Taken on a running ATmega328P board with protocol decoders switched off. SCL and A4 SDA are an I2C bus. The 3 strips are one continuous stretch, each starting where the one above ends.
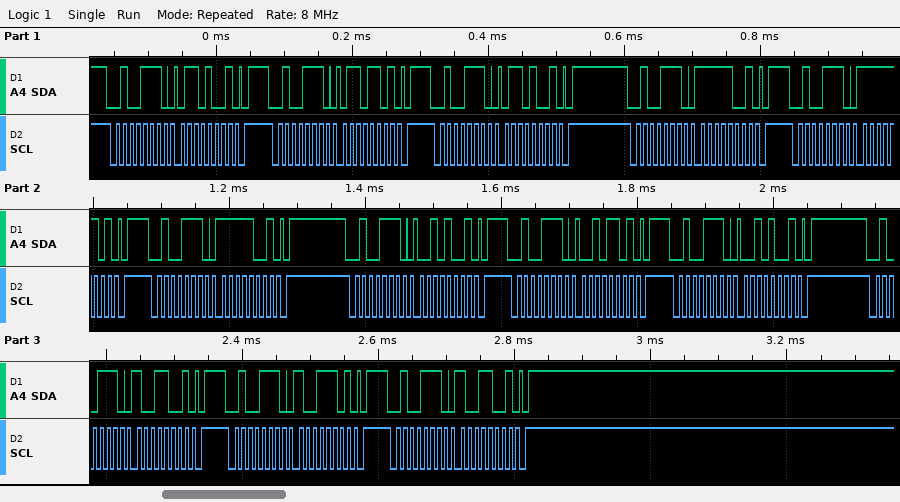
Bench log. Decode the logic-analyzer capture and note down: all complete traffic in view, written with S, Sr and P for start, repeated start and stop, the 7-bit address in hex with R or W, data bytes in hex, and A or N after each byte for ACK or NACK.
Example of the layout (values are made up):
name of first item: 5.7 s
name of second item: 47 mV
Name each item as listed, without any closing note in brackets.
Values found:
all complete traffic in view, written with S, Sr and P for start, repeated start and stop, the 7-bit address in hex with R or W, data bytes in hex, and A or N after each byte for ACK or NACK: S 27W A 69 A P S 27W A 6D A P S 27W A 69 A P S 27W A F9 A P S 27W A FD A P S 27W A F9 A P S 27W A 29 A P S 27W A 2D A P S 27W A 29 A P S 27W A 99 A P S 27W A 9D A P S 27W A 99 A P
